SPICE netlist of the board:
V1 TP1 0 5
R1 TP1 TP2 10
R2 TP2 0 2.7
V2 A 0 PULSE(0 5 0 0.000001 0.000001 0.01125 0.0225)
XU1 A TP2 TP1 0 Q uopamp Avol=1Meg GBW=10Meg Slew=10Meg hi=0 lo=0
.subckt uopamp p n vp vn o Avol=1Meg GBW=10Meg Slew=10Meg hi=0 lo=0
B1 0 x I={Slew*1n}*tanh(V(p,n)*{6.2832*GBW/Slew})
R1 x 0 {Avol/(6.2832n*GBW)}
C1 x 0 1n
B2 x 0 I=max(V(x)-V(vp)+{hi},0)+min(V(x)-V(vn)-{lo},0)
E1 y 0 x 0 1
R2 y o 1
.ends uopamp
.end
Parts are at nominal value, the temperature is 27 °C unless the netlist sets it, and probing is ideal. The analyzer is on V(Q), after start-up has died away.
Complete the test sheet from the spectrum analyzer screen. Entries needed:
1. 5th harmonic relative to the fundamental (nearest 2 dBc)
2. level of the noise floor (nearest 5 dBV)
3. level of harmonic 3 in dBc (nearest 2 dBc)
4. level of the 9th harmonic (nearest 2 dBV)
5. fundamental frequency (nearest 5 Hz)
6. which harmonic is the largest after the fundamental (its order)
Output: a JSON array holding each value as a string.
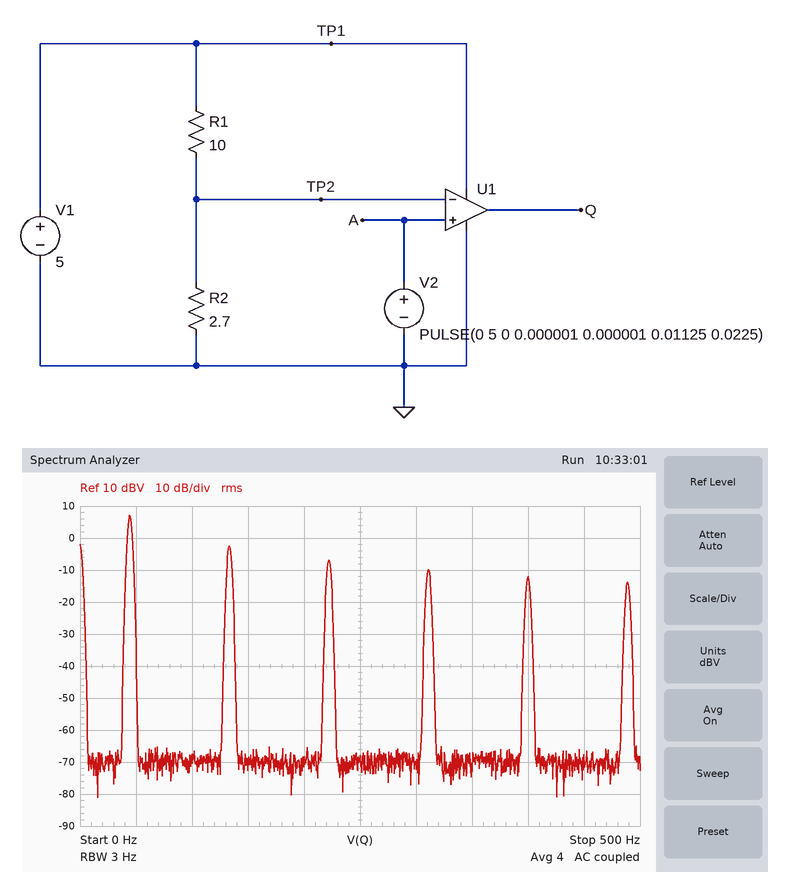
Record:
["-14 dBc", "-70 dBV", "-10 dBc", "-12 dBV", "45 Hz", "3"]
